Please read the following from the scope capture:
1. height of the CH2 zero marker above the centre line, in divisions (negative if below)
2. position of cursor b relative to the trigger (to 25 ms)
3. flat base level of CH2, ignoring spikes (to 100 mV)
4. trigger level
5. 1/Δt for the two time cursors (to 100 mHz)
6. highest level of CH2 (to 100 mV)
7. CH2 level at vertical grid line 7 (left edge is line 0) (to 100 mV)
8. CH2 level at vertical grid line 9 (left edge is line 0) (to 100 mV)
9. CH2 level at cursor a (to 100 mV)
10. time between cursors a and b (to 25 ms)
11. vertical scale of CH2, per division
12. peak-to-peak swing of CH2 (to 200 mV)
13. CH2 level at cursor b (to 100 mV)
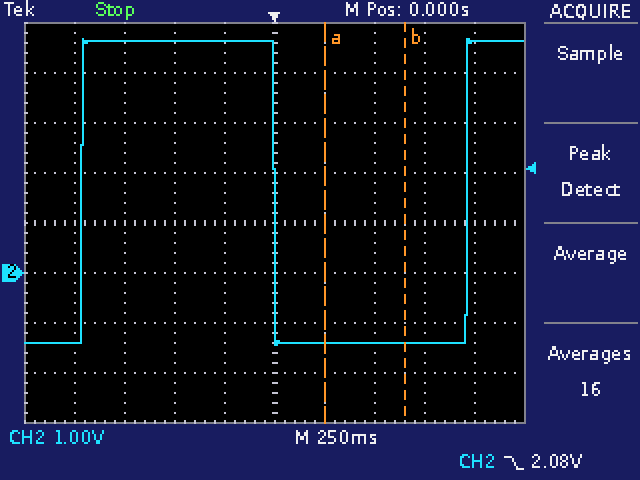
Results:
-1.0 div
+650 ms
-1.4 V
2.08 V
2.5 Hz
4.7 V
-1.4 V
4.6 V
-1.4 V
400 ms
1 V
6.2 V
-1.4 V
